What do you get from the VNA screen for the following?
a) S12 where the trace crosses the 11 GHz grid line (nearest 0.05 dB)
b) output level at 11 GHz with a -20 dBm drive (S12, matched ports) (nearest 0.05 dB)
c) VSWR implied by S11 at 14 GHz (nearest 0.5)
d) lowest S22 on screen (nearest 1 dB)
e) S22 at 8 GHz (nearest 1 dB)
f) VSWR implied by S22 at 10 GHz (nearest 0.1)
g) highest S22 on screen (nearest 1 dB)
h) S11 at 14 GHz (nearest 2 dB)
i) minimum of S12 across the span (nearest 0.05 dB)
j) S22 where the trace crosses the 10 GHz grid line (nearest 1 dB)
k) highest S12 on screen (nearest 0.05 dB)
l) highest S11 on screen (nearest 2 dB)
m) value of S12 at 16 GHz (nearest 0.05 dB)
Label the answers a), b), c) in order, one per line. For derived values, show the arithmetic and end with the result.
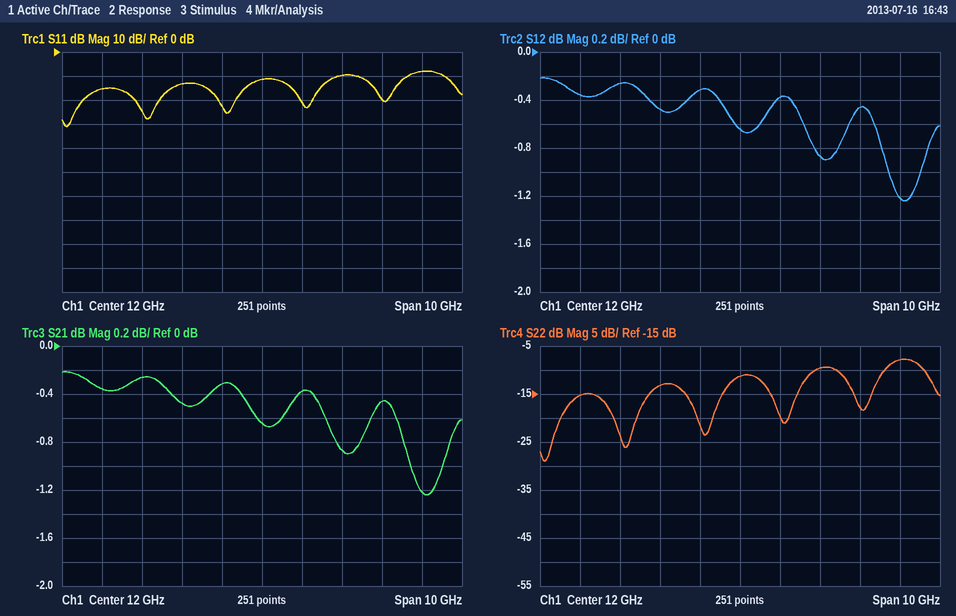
a) -0.30 dB
b) -20 dBm + (-0.30 dB) = -20.30 dBm
c) |Γ| = 10^(-10/20) = 0.3162; VSWR = (1 + 0.3162)/(1 − 0.3162) ≈ 1.92, so 2.0 to the nearest 0.5
d) -29 dB
e) -15 dB
f) |Γ| = 10^(-13/20) = 0.2239; VSWR = (1 + 0.2239)/(1 − 0.2239) ≈ 1.6
g) -8 dB
h) -10 dB
i) -1.25 dB
j) -13 dB
k) -0.20 dB
l) -8 dB
m) -1.20 dB
